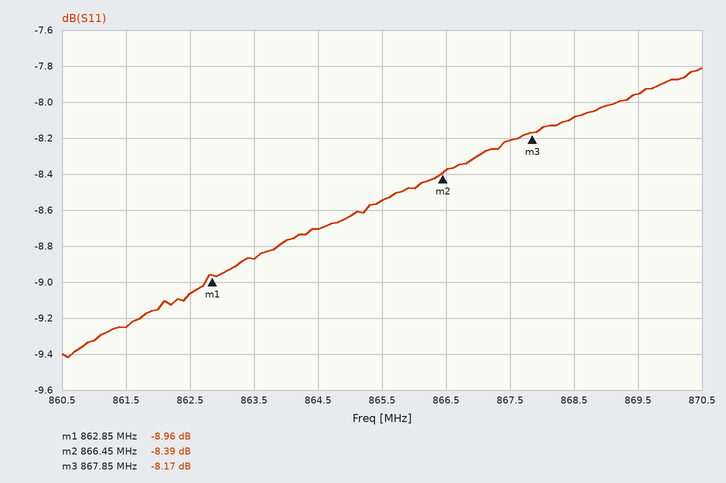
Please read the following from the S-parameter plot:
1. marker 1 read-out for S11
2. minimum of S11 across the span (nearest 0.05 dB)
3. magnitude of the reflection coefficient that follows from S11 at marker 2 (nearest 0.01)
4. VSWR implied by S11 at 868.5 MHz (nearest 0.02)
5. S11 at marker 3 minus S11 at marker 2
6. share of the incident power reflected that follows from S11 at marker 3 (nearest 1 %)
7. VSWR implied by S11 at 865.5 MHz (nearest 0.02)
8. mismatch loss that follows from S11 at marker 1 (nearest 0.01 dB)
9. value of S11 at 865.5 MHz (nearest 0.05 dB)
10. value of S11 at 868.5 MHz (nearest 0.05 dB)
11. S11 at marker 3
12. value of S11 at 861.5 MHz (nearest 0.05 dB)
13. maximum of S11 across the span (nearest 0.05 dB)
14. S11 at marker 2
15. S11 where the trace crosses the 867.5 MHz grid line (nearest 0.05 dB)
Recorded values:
-8.96 dB
-9.40 dB
0.38
2.30
0.22 dB
15 %
2.20
0.59 dB
-8.55 dB
-8.10 dB
-8.17 dB
-9.25 dB
-7.80 dB
-8.39 dB
-8.20 dB
